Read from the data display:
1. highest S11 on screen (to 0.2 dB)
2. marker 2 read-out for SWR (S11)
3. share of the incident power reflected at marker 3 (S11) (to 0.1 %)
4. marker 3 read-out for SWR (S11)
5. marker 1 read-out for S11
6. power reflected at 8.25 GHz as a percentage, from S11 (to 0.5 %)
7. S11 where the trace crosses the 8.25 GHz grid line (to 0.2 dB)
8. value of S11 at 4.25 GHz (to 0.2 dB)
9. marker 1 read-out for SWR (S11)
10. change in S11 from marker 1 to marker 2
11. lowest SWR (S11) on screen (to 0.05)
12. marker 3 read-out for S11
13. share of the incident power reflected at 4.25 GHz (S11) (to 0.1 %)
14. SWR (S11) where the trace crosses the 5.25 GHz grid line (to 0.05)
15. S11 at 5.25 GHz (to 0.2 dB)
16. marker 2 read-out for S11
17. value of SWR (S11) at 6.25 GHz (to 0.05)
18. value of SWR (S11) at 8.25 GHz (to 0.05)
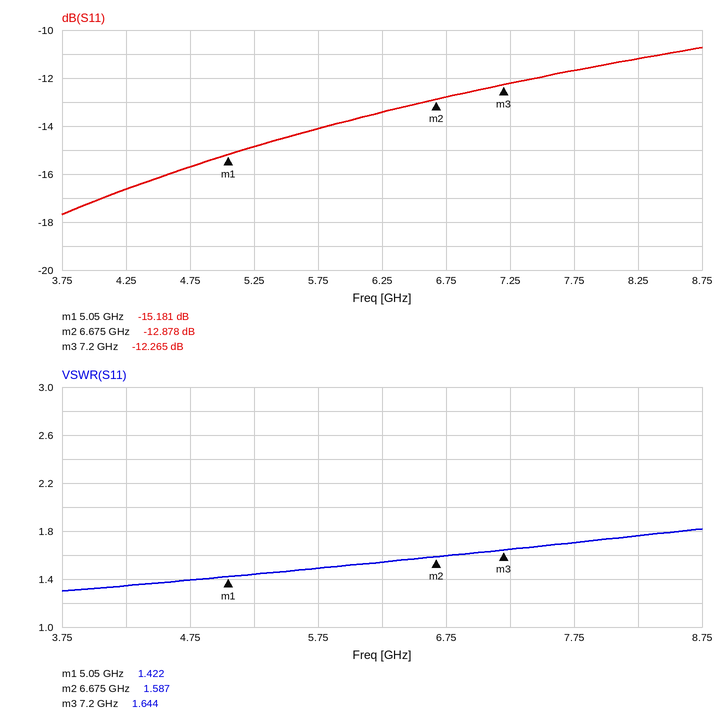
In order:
-10.8 dB
1.587
5.9 %
1.644
-15.181 dB
7.5 %
-11.2 dB
-16.6 dB
1.422
2.303 dB
1.30
-12.265 dB
2.2 %
1.45
-14.8 dB
-12.878 dB
1.55
1.75
